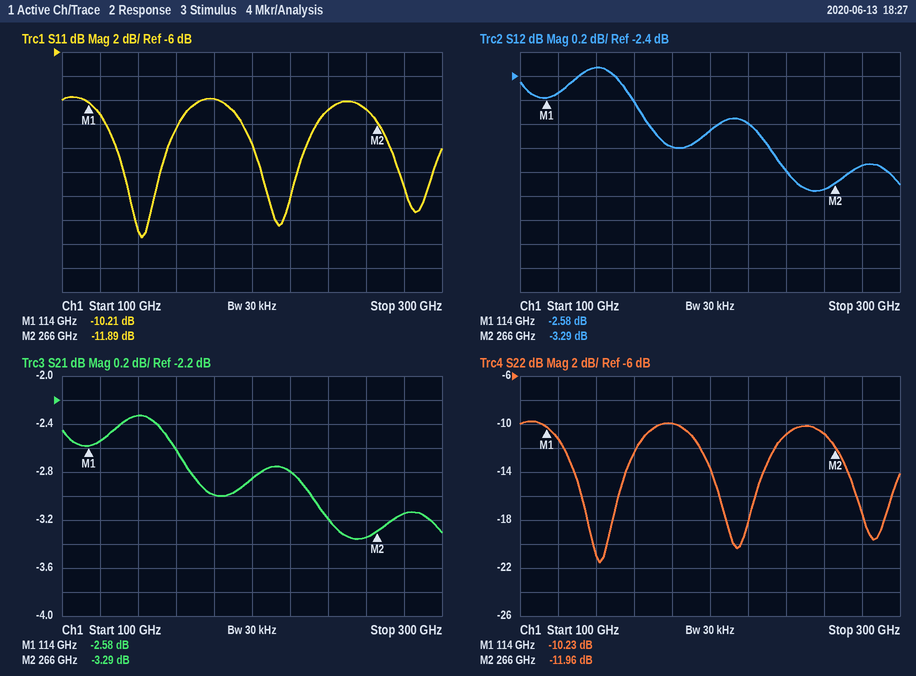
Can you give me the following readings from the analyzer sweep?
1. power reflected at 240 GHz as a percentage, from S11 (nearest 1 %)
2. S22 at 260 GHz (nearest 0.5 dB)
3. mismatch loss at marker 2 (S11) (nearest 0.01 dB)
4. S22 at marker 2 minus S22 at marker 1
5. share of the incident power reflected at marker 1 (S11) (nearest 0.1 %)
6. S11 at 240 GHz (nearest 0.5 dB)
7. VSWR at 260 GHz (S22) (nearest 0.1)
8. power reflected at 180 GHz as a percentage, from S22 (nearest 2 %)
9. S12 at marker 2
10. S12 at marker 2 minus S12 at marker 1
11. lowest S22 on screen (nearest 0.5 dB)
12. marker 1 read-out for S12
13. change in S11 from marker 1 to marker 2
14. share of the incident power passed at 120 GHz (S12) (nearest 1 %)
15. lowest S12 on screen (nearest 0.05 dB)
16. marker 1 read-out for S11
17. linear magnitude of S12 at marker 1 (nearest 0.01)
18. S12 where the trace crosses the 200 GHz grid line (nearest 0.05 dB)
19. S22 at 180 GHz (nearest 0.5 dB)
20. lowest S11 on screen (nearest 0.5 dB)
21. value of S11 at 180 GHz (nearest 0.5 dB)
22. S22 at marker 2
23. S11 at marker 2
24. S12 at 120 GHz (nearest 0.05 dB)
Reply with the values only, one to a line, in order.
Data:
8 %
-11.0 dB
0.29 dB
-1.73 dB
9.5 %
-11.0 dB
1.8
10 %
-3.29 dB
-0.71 dB
-21.5 dB
-2.58 dB
-1.68 dB
56 %
-3.35 dB
-10.21 dB
0.74
-2.85 dB
-10.0 dB
-21.5 dB
-10.0 dB
-11.96 dB
-11.89 dB
-2.55 dB
